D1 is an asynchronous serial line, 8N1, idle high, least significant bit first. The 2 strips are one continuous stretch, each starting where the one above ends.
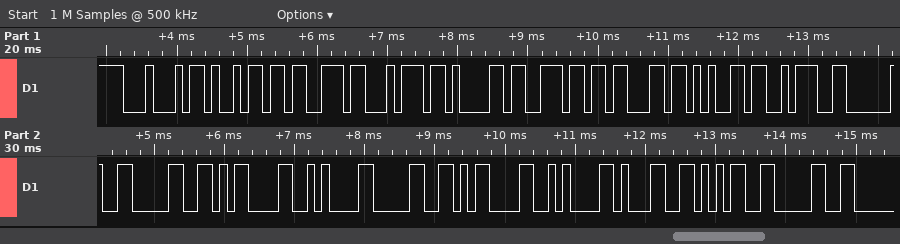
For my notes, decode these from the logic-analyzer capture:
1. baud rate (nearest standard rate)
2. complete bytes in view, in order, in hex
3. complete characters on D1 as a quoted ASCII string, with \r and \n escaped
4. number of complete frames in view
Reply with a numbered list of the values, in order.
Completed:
1. 9600 baud
2. 44 69 73 74 61 6E 63 65 3A 20 30 0D 0A 30 0D 0A 31 35 30
3. "Distance: 0\r\n0\r\n150"
4. 19
